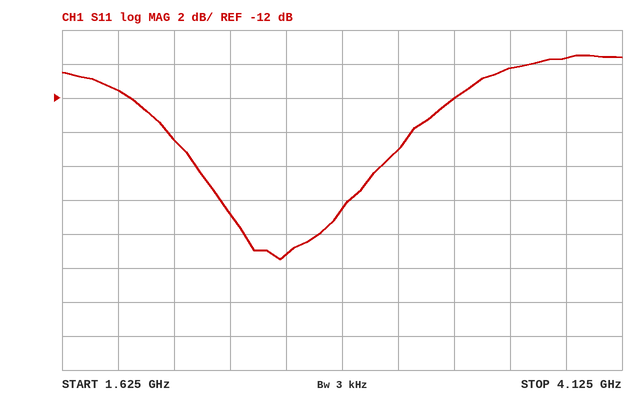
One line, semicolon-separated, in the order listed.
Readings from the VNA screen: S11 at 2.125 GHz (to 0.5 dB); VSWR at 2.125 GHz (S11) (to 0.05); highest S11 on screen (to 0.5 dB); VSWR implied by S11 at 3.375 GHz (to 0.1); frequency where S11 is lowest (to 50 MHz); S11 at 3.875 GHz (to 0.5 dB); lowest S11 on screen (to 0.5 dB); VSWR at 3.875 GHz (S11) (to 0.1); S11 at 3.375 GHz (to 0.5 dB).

-14.5 dB; 1.45; -9.5 dB; 1.7; 2.60 GHz; -9.5 dB; -21.5 dB; 2.0; -12.0 dB
